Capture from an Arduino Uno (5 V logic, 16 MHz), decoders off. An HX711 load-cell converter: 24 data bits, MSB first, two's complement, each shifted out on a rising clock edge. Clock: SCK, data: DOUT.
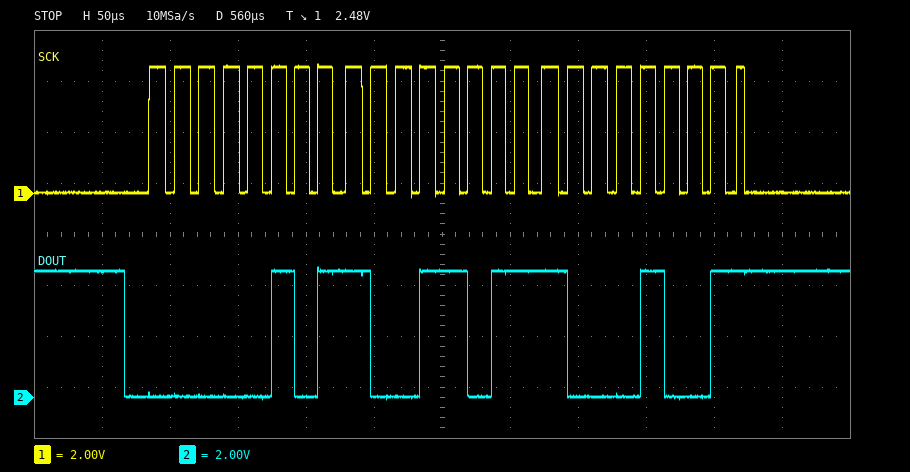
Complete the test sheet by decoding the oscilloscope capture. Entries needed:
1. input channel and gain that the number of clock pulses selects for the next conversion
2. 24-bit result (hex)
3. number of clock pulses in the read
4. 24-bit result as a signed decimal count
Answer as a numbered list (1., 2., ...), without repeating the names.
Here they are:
1. channel A, gain 128
2. 0x059B89
3. 25
4. 367497
